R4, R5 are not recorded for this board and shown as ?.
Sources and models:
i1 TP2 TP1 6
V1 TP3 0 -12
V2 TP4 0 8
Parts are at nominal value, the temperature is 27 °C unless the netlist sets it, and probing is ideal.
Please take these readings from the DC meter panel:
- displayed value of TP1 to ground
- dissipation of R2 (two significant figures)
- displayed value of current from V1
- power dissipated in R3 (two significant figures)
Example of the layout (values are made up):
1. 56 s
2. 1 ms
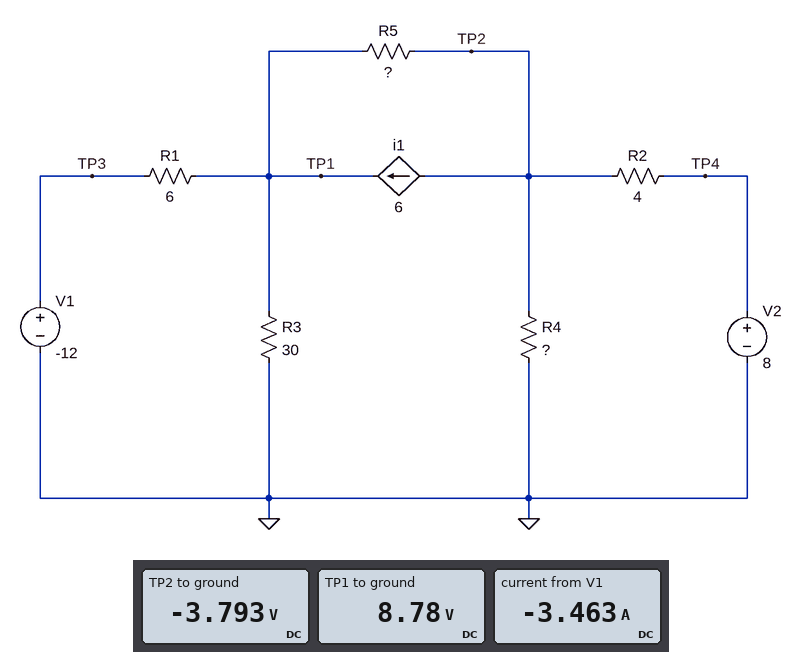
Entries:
1. 8.78 V
2. 35 W
3. -3.463 A
4. 2.6 W
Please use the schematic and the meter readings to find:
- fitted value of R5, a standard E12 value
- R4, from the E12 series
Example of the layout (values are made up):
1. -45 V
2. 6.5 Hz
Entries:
1. 5.6 Ω
2. 4.7 Ω
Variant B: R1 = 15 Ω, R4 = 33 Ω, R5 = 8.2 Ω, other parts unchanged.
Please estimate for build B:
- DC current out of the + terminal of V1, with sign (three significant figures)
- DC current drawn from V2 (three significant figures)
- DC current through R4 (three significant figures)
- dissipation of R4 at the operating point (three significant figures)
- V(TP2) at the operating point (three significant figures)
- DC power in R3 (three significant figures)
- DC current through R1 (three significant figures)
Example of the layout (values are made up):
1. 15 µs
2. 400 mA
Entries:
1. -2.24 A
2. 2.85 A
3. 103 mA
4. 352 mW
5. -3.41 V
6. 15.5 W
7. 2.24 A
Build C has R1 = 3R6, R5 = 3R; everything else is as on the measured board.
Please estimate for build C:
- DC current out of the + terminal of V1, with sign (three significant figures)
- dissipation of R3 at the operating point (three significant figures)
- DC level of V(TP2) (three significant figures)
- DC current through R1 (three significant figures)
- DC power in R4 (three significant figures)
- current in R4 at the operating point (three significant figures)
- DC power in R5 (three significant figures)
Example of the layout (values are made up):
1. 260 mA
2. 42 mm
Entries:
1. -3.88 A
2. 129 mW
3. -4.20 V
4. 3.88 A
5. 3.76 W
6. 894 mA
7. 12.7 W
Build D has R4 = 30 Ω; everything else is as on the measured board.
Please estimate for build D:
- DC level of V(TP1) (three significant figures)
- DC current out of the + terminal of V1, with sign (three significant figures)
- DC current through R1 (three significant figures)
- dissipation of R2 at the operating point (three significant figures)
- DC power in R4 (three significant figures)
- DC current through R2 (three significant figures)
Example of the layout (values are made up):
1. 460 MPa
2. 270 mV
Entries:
1. 7.93 V
2. -3.32 A
3. 3.32 A
4. 46.2 W
5. 1.04 W
6. 3.40 A
